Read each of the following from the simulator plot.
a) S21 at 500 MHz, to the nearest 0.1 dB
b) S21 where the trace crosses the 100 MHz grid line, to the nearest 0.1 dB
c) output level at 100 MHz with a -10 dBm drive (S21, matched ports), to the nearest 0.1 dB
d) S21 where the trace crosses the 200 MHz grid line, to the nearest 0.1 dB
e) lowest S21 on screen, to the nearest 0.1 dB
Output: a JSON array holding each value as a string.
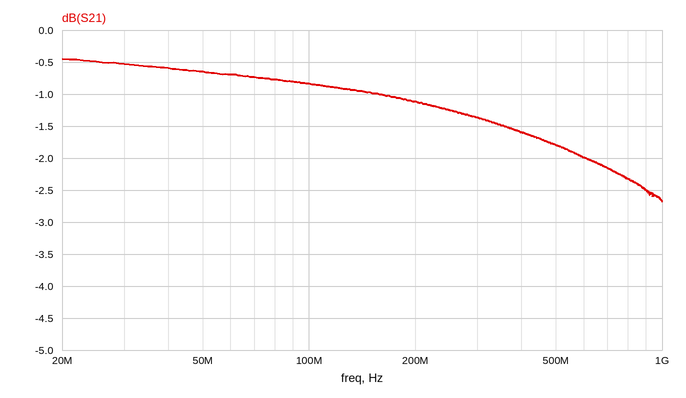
["-1.8 dB", "-0.8 dB", "-10.8 dBm", "-1.1 dB", "-2.7 dB"]
